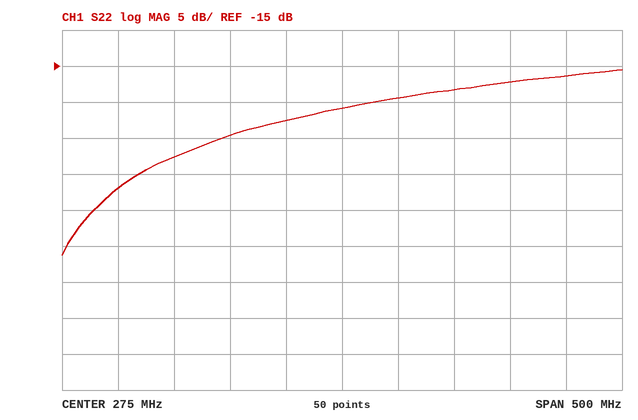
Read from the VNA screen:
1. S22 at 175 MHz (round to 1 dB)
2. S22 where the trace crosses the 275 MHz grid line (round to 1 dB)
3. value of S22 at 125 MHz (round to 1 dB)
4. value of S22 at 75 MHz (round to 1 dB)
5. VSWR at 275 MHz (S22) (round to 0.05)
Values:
-25 dB
-21 dB
-28 dB
-32 dB
1.20
